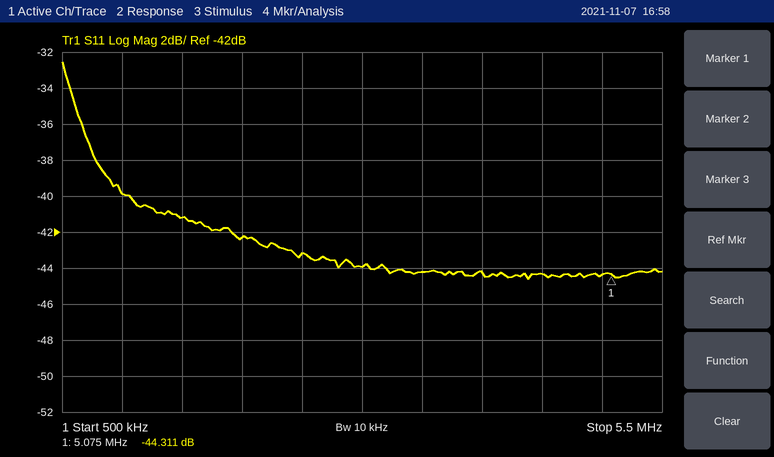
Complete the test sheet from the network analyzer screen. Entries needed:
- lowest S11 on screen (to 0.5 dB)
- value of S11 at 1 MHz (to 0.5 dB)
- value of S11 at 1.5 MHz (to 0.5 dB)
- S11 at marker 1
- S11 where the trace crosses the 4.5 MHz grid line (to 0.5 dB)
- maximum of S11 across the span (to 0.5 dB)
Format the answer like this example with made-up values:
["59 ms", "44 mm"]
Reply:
["-44.5 dB", "-40.0 dB", "-41.0 dB", "-44.311 dB", "-44.5 dB", "-32.5 dB"]
